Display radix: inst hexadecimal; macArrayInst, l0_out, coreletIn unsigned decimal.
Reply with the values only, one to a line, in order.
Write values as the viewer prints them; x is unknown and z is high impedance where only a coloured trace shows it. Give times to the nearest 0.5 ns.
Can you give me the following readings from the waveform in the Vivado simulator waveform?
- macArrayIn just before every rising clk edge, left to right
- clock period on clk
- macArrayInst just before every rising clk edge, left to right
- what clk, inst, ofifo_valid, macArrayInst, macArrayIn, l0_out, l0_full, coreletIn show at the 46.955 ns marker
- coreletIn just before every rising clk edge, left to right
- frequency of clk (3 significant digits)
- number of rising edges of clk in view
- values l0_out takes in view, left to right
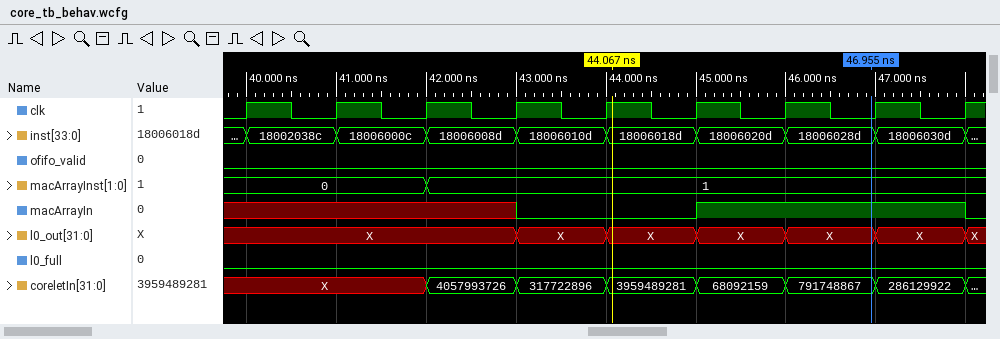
x x x x 0 0 1 1 1
1 ns
0, 0, 0, 1, 1, 1, 1, 1, 1
clk=0, inst=18006028d, ofifo_valid=0, macArrayInst=1, macArrayIn=1, l0_out=X, l0_full=0, coreletIn=791748867
X, X, X, 4057993726, 317722896, 3959489281, 68092159, 791748867, 286129922
1.00 GHz
9
X, X, X, X, X, X, X
